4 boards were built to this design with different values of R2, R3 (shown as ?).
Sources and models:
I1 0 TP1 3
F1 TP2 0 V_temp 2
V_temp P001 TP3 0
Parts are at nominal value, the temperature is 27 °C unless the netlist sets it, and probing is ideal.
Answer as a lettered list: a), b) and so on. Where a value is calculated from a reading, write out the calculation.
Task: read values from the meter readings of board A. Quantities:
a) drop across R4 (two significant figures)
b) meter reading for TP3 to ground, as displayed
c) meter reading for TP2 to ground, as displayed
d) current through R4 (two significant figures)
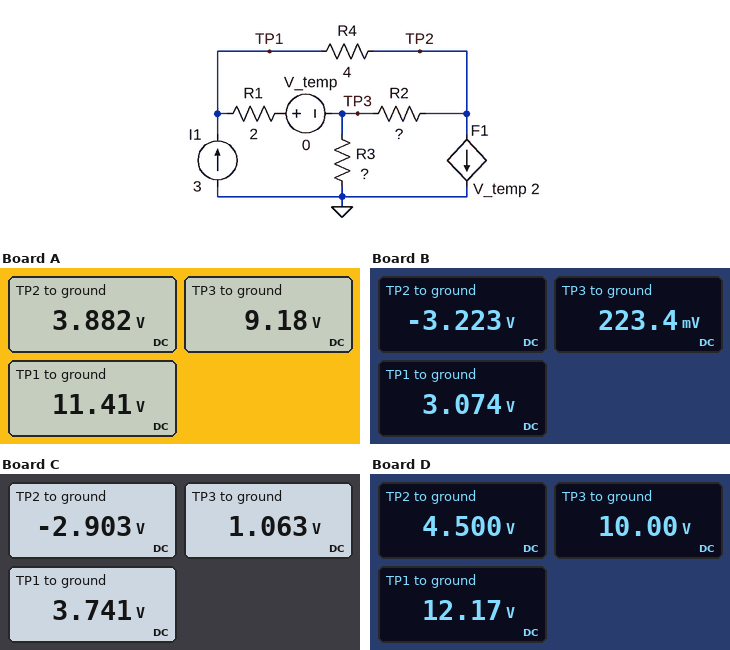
a) 11.41 V - 3.882 V = 7.5 V
b) 9.18 V
c) 3.882 V
d) (11.41 V - 3.882 V) / 4 Ω = 1.9 A
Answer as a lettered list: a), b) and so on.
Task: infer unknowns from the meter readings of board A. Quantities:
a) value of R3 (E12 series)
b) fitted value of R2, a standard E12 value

a) 12 Ω
b) 15 Ω
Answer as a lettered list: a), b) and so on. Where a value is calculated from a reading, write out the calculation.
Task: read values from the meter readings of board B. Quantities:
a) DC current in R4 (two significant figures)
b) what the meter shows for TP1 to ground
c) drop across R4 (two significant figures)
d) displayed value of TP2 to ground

a) (3.074 V - (-3.223 V)) / 4 Ω = 1.6 A
b) 3.074 V
c) 3.074 V - (-3.223 V) = 6.3 V
d) -3.223 V
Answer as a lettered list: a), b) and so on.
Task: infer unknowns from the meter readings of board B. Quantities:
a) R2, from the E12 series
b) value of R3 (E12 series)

a) 2.7 Ω
b) 1.5 Ω
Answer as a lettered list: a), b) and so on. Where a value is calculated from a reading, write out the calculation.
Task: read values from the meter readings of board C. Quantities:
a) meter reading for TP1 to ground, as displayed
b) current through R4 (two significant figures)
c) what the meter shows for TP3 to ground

a) 3.741 V
b) (3.741 V - (-2.903 V)) / 4 Ω = 1.7 A
c) 1.063 V
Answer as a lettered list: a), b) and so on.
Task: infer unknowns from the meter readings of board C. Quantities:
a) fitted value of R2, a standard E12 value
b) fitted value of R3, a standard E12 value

a) 3.9 Ω
b) 3.3 Ω
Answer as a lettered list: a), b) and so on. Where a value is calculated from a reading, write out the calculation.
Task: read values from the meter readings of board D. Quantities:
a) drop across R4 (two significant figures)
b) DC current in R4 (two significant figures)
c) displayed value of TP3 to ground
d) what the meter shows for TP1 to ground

a) 12.17 V - 4.5 V = 7.7 V
b) (12.17 V - 4.5 V) / 4 Ω = 1.9 A
c) 10.00 V
d) 12.17 V
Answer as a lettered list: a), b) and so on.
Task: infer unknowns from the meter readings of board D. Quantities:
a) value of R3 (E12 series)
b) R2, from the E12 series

a) 12 Ω
b) 22 Ω
